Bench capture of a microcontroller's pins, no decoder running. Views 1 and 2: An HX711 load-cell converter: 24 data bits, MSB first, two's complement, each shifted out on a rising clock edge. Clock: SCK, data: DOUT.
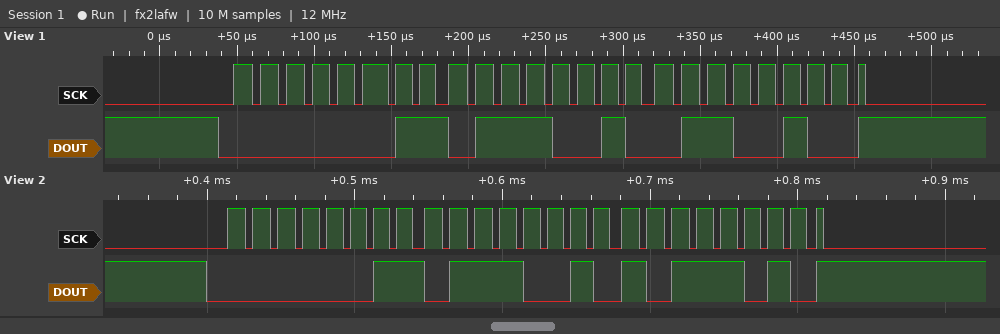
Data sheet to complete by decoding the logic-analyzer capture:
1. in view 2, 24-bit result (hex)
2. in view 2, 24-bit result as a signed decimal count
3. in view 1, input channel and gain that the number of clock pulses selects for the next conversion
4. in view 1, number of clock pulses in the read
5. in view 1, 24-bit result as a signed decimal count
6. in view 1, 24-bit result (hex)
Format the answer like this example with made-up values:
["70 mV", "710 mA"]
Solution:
["0x0372BA", "225978", "channel A, gain 128", "25", "225892", "0x037264"]
